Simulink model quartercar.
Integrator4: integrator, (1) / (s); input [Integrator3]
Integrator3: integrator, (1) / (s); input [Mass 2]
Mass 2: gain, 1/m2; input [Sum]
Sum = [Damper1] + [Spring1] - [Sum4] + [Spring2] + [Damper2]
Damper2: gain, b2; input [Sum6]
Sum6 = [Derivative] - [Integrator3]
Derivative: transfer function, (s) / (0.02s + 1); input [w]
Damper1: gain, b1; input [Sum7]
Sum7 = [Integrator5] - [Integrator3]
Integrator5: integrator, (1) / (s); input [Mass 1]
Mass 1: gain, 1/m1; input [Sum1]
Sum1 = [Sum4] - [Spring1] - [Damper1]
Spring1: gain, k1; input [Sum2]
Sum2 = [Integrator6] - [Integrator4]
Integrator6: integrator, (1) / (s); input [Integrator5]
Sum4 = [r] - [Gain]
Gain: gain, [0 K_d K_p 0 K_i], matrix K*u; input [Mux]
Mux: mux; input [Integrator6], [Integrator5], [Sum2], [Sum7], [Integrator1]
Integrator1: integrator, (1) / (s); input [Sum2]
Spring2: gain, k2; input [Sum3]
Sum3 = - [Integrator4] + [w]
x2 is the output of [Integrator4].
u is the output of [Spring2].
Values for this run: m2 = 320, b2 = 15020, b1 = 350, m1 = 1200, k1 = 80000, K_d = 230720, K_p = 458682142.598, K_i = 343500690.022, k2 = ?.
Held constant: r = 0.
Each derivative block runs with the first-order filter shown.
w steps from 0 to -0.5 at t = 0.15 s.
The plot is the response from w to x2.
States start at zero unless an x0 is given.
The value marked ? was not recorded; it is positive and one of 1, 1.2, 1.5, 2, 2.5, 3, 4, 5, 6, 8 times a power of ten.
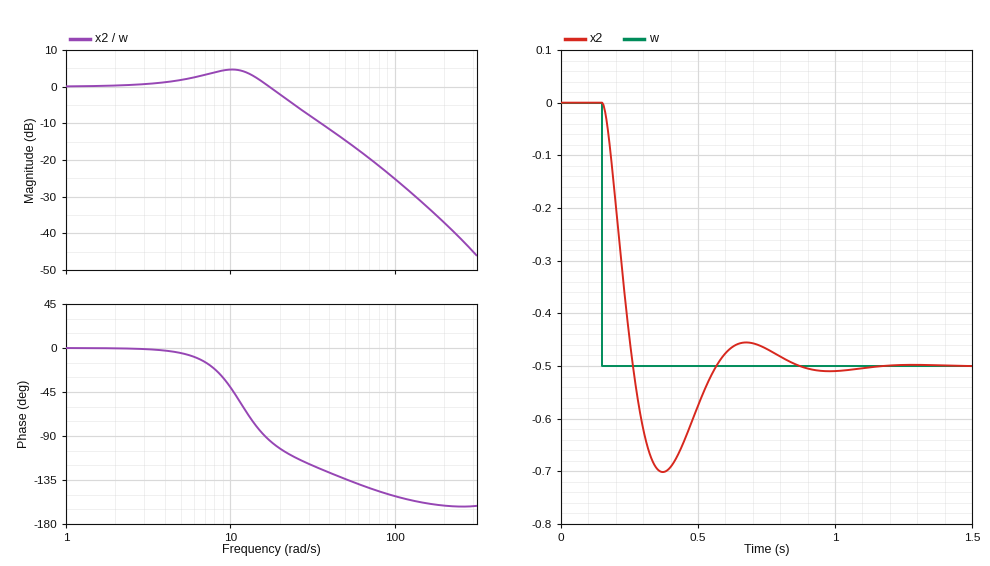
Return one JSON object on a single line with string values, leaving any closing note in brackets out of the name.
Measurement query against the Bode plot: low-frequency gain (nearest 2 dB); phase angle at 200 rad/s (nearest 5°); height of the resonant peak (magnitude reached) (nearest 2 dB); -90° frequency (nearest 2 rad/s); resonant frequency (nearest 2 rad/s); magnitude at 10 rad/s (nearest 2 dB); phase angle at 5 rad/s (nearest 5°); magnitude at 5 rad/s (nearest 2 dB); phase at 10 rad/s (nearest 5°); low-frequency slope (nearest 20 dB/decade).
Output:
{"low-frequency gain": "0 dB", "phase angle at 200 rad/s": "-160°", "height of the resonant peak (magnitude reached)": "4 dB", "-90° frequency": "16 rad/s", "resonant frequency": "10 rad/s", "magnitude at 10 rad/s": "4 dB", "phase angle at 5 rad/s": "-5°", "magnitude at 5 rad/s": "2 dB", "phase at 10 rad/s": "-40°", "low-frequency slope": "0 dB/decade"}
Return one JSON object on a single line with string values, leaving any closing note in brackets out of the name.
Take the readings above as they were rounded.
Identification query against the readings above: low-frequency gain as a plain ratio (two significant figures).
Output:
{"low-frequency gain as a plain ratio": "1.0"}
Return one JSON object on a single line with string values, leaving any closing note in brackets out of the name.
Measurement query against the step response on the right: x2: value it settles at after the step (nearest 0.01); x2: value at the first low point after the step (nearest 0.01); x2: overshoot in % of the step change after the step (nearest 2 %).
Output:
{"x2: value it settles at after the step": "-0.50", "x2: value at the first low point after the step": "-0.70", "x2: overshoot in % of the step change after the step": "40 %"}
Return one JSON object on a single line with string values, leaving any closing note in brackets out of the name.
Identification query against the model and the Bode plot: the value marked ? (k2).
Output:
{"the value marked ?": "200000"}
